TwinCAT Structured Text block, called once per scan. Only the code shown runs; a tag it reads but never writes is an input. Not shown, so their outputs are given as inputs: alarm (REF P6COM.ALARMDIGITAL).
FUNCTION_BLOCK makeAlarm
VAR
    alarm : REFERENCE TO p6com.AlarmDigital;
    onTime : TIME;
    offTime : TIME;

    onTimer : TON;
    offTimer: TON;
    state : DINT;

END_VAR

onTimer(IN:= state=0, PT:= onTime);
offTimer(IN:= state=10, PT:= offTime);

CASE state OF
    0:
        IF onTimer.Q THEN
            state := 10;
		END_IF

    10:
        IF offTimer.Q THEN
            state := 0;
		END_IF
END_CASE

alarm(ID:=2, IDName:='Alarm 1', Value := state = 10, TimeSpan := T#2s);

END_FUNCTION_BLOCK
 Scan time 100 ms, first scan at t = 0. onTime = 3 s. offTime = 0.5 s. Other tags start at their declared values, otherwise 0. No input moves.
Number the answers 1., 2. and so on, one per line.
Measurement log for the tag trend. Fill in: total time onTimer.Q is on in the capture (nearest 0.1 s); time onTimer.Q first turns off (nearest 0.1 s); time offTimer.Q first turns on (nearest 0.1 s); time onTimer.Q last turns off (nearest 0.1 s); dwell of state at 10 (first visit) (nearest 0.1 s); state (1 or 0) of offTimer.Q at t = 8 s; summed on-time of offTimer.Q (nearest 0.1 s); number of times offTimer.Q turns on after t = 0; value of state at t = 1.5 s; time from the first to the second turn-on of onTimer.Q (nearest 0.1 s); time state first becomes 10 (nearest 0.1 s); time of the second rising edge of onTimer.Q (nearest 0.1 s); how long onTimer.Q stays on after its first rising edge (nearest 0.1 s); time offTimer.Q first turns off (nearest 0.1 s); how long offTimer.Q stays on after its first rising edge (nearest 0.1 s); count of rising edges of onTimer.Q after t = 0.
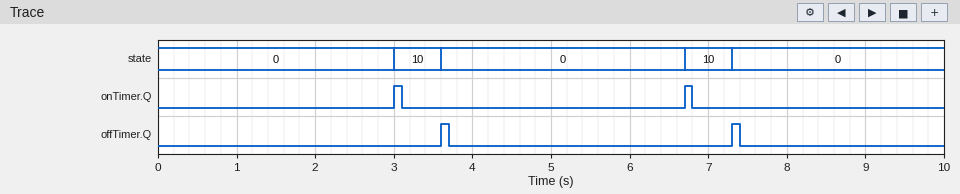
1. 0.2 s
2. 3.1 s
3. 3.6 s
4. 6.8 s
5. 0.6 s
6. 0
7. 0.2 s
8. 2
9. 0
10. 3.7 s
11. 3.0 s
12. 6.7 s
13. 0.1 s
14. 3.7 s
15. 0.1 s
16. 2
